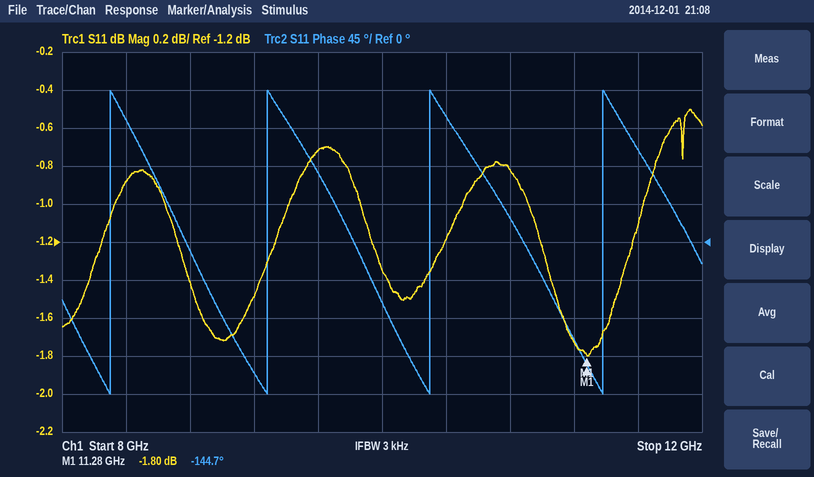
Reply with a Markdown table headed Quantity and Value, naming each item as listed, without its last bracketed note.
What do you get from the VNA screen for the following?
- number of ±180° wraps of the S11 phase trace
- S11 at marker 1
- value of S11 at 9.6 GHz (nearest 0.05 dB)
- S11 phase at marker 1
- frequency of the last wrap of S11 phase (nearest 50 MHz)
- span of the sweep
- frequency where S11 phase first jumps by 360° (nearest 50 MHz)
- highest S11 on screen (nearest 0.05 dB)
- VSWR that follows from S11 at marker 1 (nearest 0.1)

| Quantity | Value |
|---|---|
| number of ±180° wraps of the S11 phase trace | 4 |
| S11 at marker 1 | -1.80 dB |
| value of S11 at 9.6 GHz | -0.70 dB |
| S11 phase at marker 1 | -144.7° |
| frequency of the last wrap of S11 phase | 11.40 GHz |
| span of the sweep | 4 GHz |
| frequency where S11 phase first jumps by 360° | 8.30 GHz |
| highest S11 on screen | -0.50 dB |
| VSWR that follows from S11 at marker 1 | 9.7 |
